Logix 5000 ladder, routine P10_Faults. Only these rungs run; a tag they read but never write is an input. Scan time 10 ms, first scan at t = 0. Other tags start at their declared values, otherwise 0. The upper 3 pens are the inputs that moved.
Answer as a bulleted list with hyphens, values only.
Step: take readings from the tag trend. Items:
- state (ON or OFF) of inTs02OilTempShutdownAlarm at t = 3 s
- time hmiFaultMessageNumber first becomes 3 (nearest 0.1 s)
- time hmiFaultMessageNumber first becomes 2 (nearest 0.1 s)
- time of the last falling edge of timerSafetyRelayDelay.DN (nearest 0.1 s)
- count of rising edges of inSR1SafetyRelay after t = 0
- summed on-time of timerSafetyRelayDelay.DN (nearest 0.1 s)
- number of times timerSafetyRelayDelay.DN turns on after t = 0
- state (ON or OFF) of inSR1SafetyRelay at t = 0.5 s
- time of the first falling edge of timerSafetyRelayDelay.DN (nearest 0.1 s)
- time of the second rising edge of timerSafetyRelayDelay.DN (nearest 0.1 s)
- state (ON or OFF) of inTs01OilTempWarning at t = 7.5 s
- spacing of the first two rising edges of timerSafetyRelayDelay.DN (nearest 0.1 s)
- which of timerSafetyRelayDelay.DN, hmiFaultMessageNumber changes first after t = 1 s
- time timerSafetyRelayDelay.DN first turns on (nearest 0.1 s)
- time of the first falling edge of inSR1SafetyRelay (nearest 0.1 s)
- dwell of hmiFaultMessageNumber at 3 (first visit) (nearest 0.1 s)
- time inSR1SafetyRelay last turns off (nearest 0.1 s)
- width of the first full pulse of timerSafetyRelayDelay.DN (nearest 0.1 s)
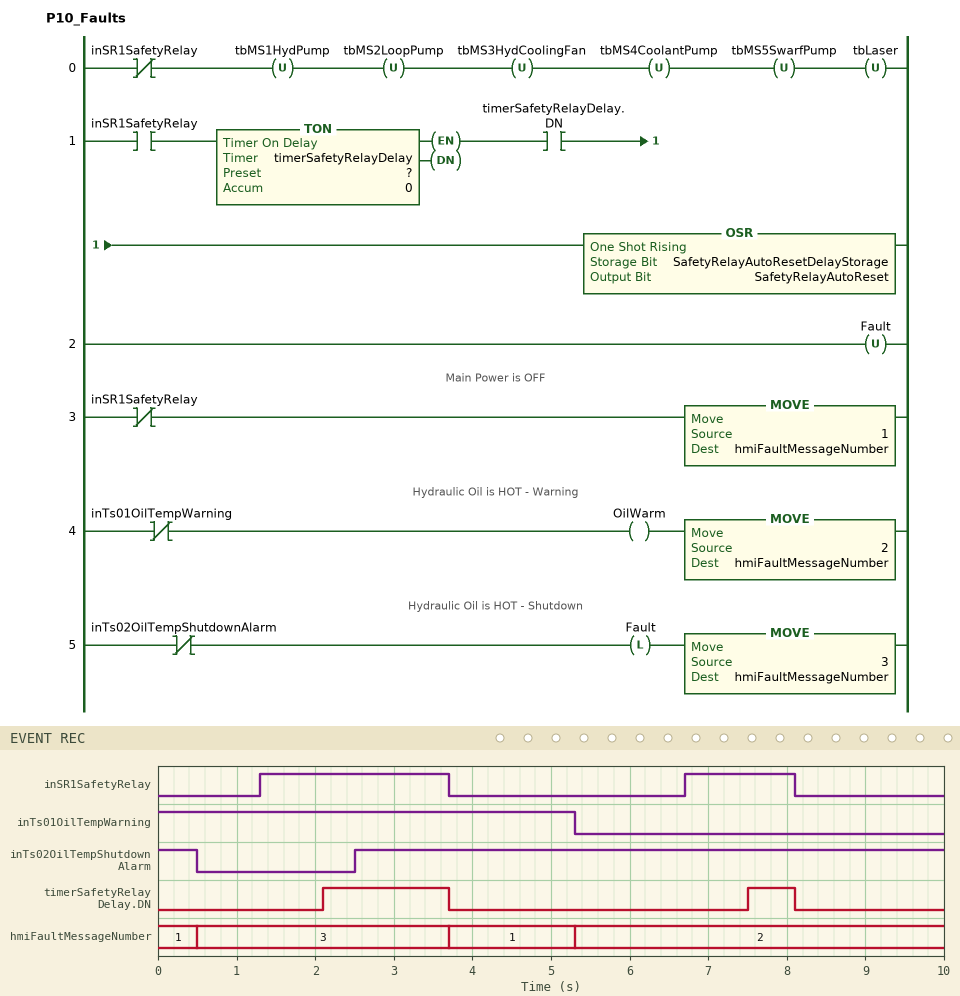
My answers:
- ON
- 0.5 s
- 5.3 s
- 8.1 s
- 2
- 2.2 s
- 2
- OFF
- 3.7 s
- 7.5 s
- OFF
- 5.4 s
- timerSafetyRelayDelay.DN
- 2.1 s
- 3.7 s
- 3.2 s
- 8.1 s
- 1.6 s
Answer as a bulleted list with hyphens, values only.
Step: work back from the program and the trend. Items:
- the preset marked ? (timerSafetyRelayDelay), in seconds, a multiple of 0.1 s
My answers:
- 0.8 s
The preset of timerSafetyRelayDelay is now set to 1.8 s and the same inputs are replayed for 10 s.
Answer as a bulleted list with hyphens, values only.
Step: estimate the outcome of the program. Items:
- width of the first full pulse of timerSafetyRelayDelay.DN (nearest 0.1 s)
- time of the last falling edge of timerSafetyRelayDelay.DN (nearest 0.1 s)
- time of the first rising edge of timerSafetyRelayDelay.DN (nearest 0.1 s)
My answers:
- 0.6 s
- 3.7 s
- 3.1 s
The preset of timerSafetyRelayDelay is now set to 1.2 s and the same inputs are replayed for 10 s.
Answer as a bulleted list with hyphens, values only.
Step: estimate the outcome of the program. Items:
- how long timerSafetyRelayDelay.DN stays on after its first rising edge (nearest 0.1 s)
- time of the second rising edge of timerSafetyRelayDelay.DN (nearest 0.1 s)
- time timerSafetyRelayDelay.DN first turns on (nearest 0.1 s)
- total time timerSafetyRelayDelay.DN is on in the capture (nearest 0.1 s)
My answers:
- 1.2 s
- 7.9 s
- 2.5 s
- 1.4 s
